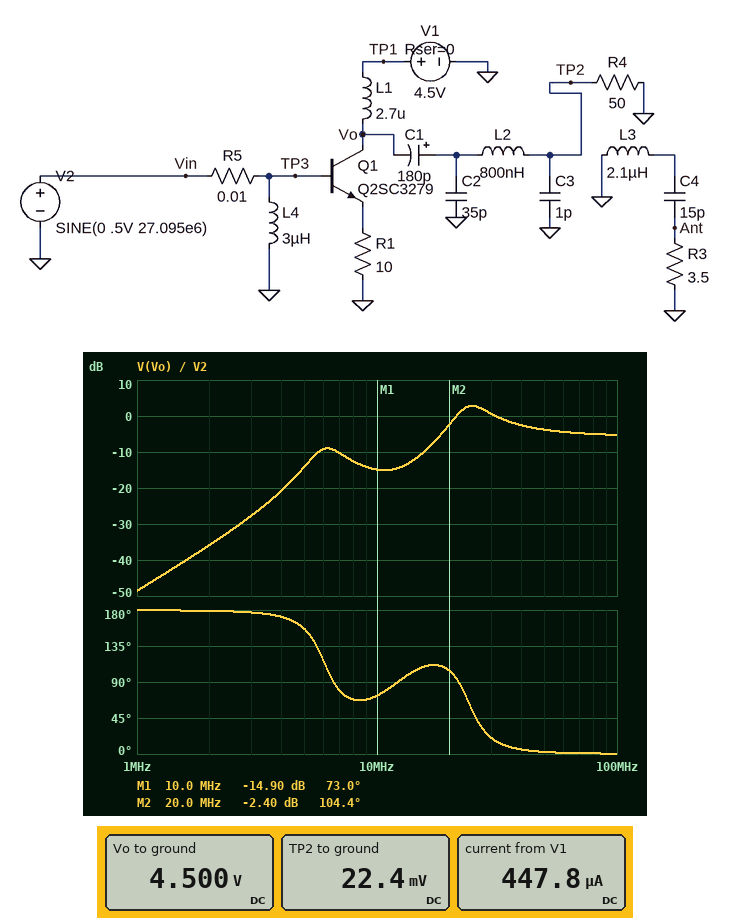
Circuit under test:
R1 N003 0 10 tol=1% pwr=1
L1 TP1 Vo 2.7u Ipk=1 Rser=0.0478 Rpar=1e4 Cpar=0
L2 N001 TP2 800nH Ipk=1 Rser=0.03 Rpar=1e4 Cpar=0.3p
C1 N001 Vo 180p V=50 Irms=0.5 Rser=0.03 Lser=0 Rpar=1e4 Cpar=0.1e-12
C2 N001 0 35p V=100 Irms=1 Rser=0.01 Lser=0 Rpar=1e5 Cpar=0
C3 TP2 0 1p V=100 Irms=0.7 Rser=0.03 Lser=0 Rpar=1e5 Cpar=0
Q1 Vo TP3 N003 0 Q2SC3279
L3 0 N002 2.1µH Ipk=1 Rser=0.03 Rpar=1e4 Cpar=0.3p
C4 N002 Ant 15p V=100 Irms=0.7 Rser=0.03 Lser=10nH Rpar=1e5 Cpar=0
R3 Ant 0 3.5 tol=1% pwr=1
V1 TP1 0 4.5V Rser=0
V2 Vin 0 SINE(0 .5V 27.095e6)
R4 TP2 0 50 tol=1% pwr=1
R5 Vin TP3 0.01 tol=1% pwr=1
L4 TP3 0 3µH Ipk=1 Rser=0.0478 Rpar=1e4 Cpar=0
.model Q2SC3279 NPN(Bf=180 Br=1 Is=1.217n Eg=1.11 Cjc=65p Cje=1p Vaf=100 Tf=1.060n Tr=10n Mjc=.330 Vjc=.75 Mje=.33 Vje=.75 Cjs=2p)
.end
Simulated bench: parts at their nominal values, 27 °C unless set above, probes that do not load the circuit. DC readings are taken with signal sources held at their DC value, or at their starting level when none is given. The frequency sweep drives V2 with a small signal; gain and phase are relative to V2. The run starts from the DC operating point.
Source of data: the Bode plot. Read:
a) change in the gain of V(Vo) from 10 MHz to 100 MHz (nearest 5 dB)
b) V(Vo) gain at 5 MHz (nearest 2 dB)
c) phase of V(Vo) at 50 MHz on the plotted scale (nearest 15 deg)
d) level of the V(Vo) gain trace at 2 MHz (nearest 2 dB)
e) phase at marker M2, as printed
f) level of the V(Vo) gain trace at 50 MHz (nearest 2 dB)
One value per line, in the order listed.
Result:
10 dB
-14 dB
0 deg
-36 dB
104.4 deg
-4 dB
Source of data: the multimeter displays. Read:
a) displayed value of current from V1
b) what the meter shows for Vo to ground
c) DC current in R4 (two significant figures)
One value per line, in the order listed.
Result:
447.8 µA
4.500 V
450 µA
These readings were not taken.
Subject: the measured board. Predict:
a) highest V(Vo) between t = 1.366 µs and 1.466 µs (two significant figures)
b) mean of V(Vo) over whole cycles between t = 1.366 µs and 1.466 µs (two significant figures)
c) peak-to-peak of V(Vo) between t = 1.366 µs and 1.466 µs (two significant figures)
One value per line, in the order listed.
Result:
5.4 V
4.5 V
1.8 V
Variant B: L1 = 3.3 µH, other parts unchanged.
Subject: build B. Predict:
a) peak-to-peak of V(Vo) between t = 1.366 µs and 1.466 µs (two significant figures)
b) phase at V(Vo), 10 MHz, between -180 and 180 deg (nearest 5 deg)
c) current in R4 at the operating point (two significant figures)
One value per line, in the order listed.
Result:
1.7 V
70 deg
450 µA
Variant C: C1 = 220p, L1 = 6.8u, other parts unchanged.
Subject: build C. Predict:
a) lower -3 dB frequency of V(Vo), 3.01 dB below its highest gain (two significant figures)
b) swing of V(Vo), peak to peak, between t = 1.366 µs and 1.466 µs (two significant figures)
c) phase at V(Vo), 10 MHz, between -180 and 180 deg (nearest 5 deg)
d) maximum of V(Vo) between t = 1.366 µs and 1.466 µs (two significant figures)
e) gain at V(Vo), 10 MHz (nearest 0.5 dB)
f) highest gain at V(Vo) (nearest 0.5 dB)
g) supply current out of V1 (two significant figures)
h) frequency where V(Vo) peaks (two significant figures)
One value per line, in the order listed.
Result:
20 MHz
1.5 V
70 deg
5.3 V
-17.0 dB
1.0 dB
450 µA
24 MHz
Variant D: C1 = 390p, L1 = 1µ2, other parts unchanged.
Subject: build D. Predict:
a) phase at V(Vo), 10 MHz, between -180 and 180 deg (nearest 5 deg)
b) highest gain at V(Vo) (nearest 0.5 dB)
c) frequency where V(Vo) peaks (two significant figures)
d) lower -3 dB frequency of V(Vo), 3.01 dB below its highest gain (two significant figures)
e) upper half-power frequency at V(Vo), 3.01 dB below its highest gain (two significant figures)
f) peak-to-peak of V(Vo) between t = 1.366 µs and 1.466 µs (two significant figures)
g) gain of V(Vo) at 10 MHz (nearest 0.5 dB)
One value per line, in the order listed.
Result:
130 deg
6.5 dB
27 MHz
24 MHz
31 MHz
3.0 V
-19.5 dB
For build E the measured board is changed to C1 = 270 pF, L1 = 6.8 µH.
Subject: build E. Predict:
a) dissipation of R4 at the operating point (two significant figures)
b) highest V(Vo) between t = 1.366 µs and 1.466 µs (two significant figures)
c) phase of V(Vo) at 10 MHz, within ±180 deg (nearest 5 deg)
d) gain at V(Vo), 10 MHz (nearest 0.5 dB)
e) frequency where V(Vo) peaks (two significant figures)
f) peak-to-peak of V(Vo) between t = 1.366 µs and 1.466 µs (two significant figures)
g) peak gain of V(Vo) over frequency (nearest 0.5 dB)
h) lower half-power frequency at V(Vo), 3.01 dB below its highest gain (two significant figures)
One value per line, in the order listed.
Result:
10 µW
5.3 V
80 deg
-17.5 dB
24 MHz
1.5 V
1.5 dB
20 MHz
